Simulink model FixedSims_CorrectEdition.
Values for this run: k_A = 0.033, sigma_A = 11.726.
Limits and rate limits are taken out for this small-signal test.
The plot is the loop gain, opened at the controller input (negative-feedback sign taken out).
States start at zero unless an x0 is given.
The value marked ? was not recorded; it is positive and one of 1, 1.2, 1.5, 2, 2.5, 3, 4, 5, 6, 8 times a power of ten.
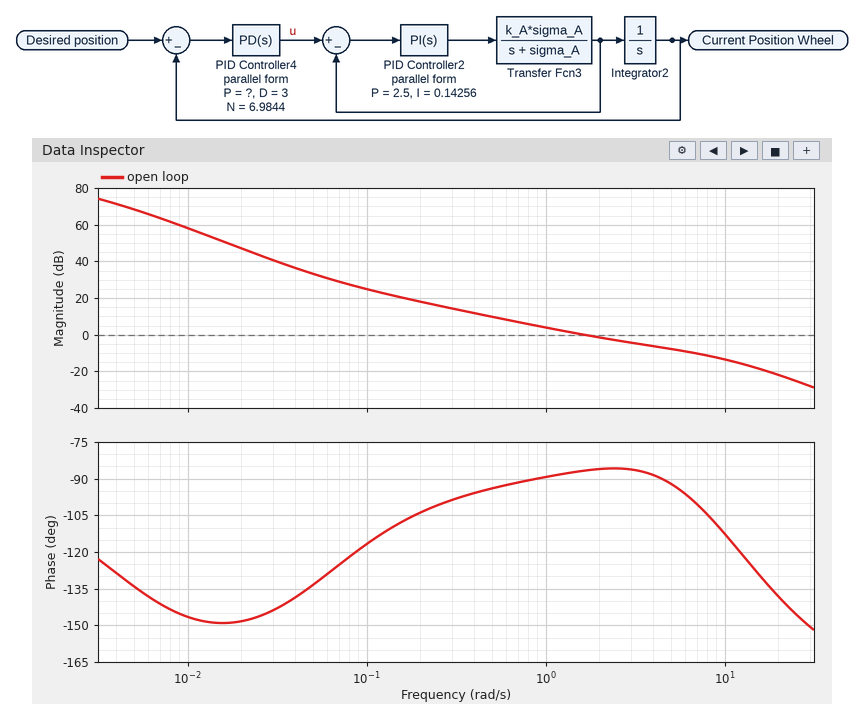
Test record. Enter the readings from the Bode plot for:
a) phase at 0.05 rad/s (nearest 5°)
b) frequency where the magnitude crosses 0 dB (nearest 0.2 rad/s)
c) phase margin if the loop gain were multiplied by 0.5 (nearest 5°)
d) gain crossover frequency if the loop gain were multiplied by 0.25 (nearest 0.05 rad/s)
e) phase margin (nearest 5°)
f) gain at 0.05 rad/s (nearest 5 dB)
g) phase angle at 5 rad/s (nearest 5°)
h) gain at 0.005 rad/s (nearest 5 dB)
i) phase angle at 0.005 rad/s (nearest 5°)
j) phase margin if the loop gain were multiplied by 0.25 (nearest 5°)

-135°
1.6 rad/s
90°
0.40 rad/s
95°
35 dB
-90°
70 dB
-135°
85°
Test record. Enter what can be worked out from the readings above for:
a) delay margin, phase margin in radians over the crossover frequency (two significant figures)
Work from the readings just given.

1.0 s
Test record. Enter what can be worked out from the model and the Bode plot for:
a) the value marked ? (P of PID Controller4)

20
